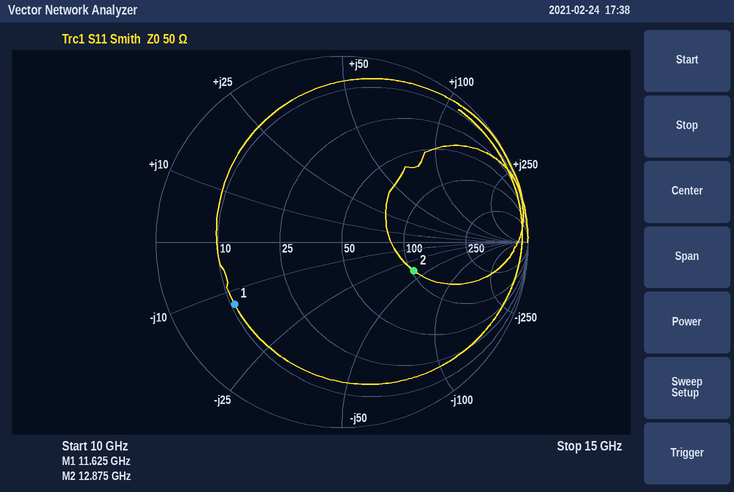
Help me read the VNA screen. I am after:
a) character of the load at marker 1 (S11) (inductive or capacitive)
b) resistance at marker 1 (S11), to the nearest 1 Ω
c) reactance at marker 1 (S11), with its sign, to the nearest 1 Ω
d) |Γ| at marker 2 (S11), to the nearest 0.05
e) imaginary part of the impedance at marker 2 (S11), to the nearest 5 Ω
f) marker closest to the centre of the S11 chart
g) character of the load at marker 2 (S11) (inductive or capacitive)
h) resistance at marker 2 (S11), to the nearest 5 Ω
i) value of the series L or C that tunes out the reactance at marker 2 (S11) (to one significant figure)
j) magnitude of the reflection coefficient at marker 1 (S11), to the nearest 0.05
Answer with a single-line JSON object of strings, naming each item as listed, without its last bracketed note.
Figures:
{"character of the load at marker 1 (S11)": "capacitive", "resistance at marker 1 (S11), to the nearest 1 Ω": "11 Ω", "reactance at marker 1 (S11), with its sign, to the nearest 1 Ω": "-13 Ω", "|Γ| at marker 2 (S11), to the nearest 0.05": "0.40", "imaginary part of the impedance at marker 2 (S11), to the nearest 5 Ω": "-40 Ω", "marker closest to the centre of the S11 chart": "marker 2", "character of the load at marker 2 (S11)": "capacitive", "resistance at marker 2 (S11), to the nearest 5 Ω": "105 Ω", "value of the series L or C that tunes out the reactance at marker 2 (S11)": "500 pH", "magnitude of the reflection coefficient at marker 1 (S11), to the nearest 0.05": "0.65"}
